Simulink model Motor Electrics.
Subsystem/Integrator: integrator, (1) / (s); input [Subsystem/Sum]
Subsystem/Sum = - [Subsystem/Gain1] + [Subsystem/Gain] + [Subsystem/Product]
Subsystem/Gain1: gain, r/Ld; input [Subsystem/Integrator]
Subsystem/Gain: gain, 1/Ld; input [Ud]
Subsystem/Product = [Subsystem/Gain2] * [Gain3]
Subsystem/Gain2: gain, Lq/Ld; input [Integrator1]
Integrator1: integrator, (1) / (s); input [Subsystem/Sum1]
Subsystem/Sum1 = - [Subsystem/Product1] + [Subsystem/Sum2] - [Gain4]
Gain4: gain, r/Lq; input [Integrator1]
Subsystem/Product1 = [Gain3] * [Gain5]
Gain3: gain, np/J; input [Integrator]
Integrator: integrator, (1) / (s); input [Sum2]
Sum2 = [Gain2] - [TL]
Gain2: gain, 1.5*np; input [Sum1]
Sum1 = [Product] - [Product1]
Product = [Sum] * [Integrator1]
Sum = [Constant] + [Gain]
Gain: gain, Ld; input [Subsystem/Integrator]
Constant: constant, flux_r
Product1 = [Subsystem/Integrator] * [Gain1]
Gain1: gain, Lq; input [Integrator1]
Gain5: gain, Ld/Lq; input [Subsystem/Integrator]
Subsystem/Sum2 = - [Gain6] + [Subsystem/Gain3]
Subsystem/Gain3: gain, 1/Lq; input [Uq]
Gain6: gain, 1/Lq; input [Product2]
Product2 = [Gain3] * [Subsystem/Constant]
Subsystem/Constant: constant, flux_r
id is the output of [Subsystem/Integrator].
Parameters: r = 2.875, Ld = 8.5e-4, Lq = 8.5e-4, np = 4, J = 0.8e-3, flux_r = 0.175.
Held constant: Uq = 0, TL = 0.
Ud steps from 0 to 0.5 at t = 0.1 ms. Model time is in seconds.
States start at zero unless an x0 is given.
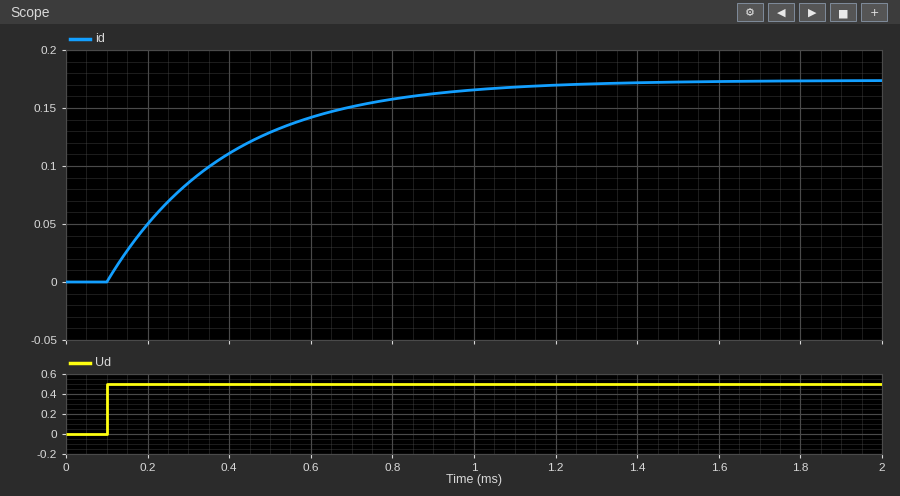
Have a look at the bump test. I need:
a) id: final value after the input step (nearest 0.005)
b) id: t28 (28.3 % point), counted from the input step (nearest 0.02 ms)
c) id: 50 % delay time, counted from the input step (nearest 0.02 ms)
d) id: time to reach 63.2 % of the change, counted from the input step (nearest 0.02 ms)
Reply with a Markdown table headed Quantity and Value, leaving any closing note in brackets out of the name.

| Quantity | Value |
|---|---|
| id: final value after the input step | 0.175 |
| id: t28 (28.3 % point), counted from the input step | 0.10 ms |
| id: 50 % delay time, counted from the input step | 0.20 ms |
| id: time to reach 63.2 % of the change, counted from the input step | 0.30 ms |
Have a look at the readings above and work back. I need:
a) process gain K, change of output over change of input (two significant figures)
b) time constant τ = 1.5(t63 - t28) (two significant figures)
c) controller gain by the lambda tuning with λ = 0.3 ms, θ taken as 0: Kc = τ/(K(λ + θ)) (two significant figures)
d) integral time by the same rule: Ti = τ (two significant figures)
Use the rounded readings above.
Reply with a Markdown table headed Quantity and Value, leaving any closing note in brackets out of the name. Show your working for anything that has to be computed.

| Quantity | Value |
|---|---|
| process gain K, change of output over change of input | (0.175 - 0) / 0.5 = 0.35 |
| time constant τ = 1.5(t63 - t28) | 1.5 × (0.3 - 0.1) = 0.30 ms |
| controller gain by the lambda tuning with λ = 0.3 ms, θ taken as 0: Kc = τ/(K(λ + θ)) | 0.3 / (0.35 × (0.3 + 0)) = 2.9 |
| integral time by the same rule: Ti = τ | 0.30 ms |
